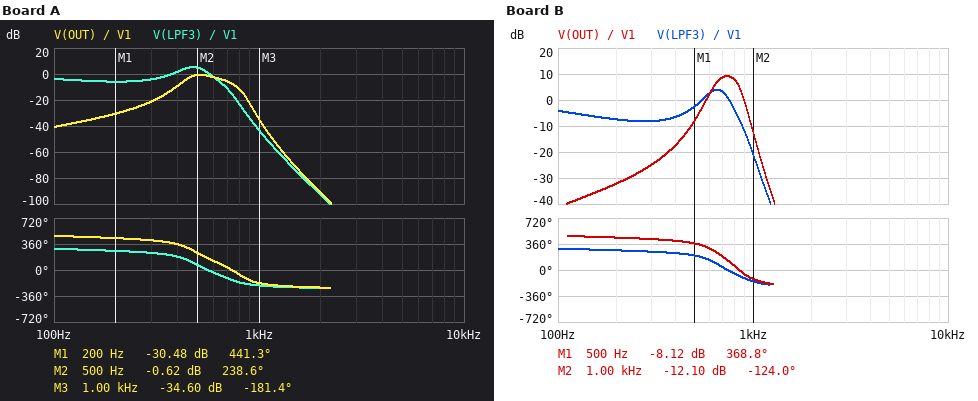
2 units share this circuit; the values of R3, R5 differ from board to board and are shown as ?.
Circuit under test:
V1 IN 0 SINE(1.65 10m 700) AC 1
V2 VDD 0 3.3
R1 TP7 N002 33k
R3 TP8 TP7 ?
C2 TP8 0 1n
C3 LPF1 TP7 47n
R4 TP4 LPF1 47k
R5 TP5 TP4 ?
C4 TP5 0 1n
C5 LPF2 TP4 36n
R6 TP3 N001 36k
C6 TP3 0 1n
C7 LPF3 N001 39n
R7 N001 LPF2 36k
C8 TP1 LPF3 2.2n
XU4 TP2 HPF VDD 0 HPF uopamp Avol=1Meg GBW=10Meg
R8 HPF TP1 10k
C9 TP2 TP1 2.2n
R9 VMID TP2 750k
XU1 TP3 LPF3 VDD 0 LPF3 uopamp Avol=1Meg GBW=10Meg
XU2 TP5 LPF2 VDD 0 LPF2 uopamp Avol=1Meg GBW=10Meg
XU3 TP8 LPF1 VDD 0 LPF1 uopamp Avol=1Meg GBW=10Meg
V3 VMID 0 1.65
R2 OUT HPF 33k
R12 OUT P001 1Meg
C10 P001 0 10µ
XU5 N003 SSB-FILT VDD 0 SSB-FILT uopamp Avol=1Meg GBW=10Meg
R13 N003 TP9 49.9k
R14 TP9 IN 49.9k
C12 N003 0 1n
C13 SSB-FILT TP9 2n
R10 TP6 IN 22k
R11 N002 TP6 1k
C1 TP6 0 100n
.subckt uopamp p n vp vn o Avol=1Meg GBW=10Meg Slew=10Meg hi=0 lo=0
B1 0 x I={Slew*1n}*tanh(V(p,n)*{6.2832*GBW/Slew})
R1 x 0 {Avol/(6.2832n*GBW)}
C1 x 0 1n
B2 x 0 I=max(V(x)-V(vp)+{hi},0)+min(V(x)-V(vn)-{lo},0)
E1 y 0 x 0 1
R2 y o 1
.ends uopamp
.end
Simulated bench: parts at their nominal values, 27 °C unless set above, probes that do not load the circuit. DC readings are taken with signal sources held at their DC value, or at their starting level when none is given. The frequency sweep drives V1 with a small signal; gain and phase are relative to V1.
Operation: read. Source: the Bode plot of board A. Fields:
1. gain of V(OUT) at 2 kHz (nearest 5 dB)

-90 dB
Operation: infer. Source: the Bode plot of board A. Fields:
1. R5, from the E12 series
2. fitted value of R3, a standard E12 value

68 kΩ
56 kΩ
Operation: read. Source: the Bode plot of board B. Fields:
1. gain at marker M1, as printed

-8.12 dB
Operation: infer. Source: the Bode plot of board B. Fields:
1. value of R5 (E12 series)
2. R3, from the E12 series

18 kΩ
39 kΩ
